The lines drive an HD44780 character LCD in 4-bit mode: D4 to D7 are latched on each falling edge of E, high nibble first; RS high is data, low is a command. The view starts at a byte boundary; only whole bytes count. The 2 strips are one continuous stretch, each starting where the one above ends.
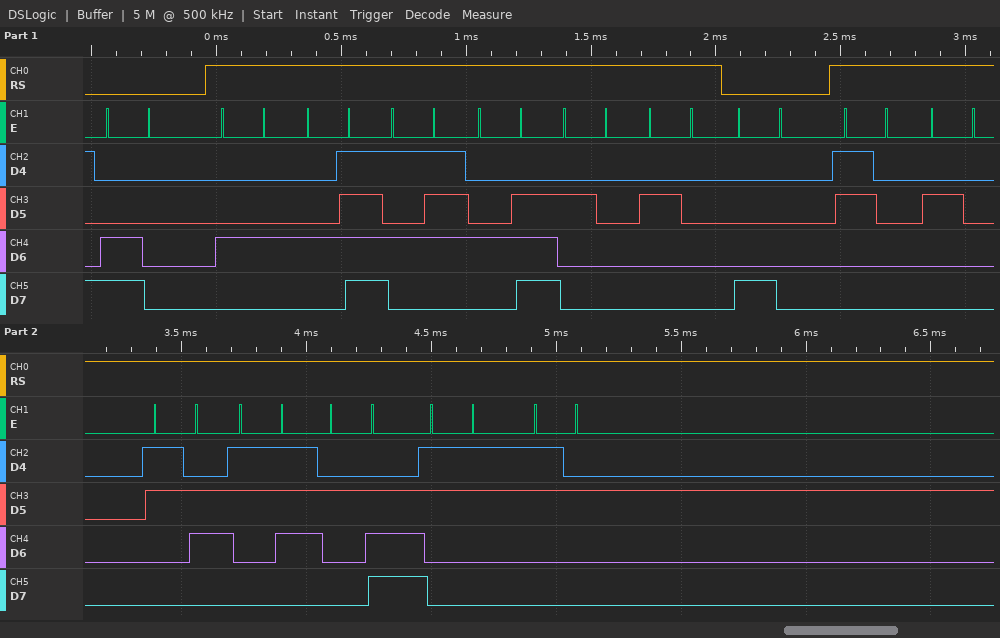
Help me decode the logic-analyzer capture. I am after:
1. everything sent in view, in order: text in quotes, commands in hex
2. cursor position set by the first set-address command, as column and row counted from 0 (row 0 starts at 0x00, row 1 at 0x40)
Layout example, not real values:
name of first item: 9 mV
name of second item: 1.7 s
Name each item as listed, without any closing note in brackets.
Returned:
everything sent in view, in order: text in quotes, commands in hex: 0xC0 "DOWN  " 0x80 "0 67.32"
cursor position set by the first set-address command, as column and row counted from 0: column 0, row 1
